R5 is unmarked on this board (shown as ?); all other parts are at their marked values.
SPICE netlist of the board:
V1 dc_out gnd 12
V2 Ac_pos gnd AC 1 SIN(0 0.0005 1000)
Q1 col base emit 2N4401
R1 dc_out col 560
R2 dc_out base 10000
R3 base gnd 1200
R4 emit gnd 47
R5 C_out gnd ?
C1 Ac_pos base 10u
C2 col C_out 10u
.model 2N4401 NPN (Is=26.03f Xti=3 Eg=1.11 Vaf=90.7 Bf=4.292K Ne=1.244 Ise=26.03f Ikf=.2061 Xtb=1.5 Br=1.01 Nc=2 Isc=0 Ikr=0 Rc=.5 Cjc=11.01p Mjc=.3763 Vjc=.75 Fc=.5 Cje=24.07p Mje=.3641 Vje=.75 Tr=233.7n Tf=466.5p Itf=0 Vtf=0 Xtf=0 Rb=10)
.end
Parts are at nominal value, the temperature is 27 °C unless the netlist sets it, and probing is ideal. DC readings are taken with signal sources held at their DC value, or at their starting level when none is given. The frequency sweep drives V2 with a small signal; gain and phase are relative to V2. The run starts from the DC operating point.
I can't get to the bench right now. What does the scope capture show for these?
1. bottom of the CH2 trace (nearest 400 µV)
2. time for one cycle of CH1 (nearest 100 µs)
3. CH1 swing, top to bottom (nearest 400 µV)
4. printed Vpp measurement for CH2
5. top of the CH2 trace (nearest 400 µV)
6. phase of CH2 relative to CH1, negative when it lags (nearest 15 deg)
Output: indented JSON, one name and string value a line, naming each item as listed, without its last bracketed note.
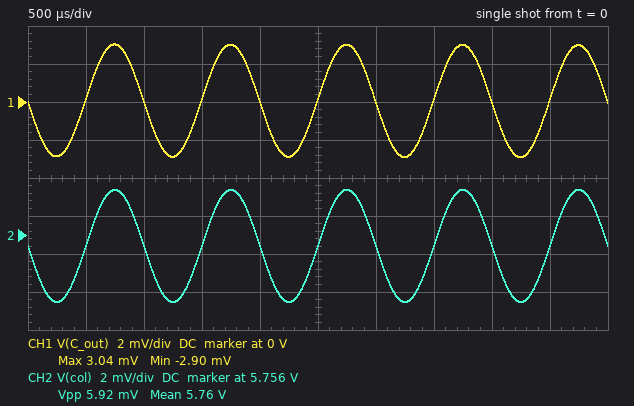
{
  "bottom of the CH2 trace": "5.7524 V",
  "time for one cycle of CH1": "1.0 ms",
  "CH1 swing, top to bottom": "6.0 mV",
  "printed Vpp measurement for CH2": "5.92 mV",
  "top of the CH2 trace": "5.7584 V",
  "phase of CH2 relative to CH1, negative when it lags": "0 deg"
}
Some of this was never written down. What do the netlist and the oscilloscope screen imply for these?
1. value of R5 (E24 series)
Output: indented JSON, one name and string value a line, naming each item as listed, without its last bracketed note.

{
  "value of R5": "620 Ω"
}
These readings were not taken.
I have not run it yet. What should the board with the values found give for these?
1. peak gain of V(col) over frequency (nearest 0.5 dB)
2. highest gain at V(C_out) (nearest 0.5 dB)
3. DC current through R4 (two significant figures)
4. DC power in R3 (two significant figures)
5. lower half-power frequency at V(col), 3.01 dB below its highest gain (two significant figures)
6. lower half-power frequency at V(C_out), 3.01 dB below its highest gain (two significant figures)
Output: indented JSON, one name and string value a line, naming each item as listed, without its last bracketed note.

{
  "peak gain of V(col) over frequency": "16.0 dB",
  "highest gain at V(C_out)": "15.5 dB",
  "DC current through R4": "11 mA",
  "DC power in R3": "1.2 mW",
  "lower half-power frequency at V(col), 3.01 dB below its highest gain": "7.9 Hz",
  "lower half-power frequency at V(C_out), 3.01 dB below its highest gain": "23 Hz"
}
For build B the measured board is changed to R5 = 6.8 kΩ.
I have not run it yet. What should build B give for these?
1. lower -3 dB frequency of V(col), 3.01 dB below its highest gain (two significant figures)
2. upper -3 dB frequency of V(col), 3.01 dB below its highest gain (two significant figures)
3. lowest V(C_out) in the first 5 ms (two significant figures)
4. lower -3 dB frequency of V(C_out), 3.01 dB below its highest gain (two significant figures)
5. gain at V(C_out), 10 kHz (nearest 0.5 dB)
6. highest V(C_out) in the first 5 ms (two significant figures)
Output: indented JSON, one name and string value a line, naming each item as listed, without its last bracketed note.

{
  "lower -3 dB frequency of V(col), 3.01 dB below its highest gain": "16 Hz",
  "upper -3 dB frequency of V(col), 3.01 dB below its highest gain": "46 MHz",
  "lowest V(C_out) in the first 5 ms": "-5.1 mV",
  "lower -3 dB frequency of V(C_out), 3.01 dB below its highest gain": "17 Hz",
  "gain at V(C_out), 10 kHz": "20.5 dB",
  "highest V(C_out) in the first 5 ms": "5.3 mV"
}
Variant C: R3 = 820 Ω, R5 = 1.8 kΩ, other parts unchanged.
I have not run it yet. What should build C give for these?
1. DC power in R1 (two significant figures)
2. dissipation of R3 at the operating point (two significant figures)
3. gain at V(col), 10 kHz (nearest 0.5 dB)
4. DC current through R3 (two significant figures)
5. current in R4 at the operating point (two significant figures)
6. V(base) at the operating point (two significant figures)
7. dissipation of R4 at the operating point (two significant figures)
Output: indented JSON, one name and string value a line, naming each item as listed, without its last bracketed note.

{
  "DC power in R1": "12 mW",
  "dissipation of R3 at the operating point": "960 µW",
  "gain at V(col), 10 kHz": "18.0 dB",
  "DC current through R3": "1.1 mA",
  "current in R4 at the operating point": "4.7 mA",
  "V(base) at the operating point": "890 mV",
  "dissipation of R4 at the operating point": "1.0 mW"
}
